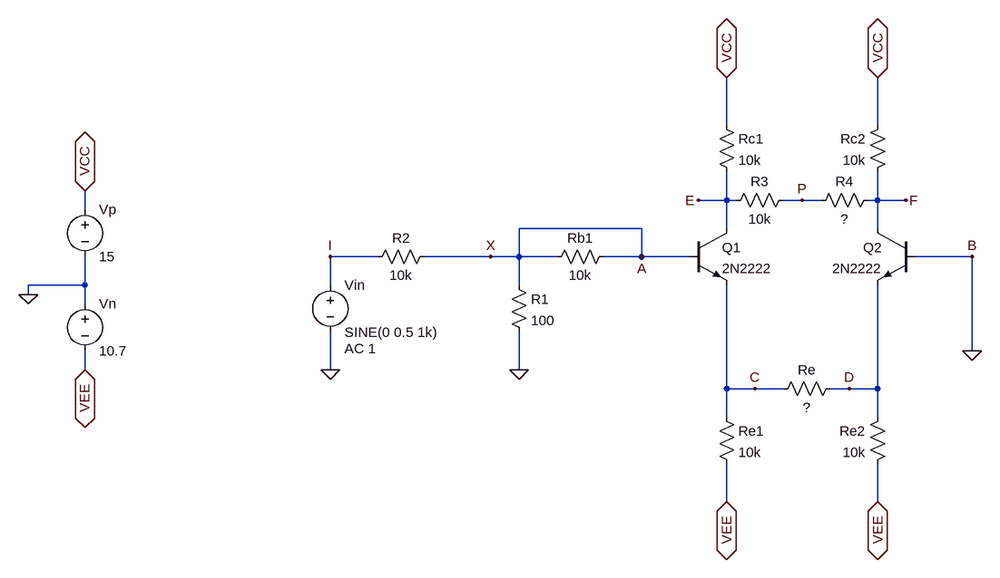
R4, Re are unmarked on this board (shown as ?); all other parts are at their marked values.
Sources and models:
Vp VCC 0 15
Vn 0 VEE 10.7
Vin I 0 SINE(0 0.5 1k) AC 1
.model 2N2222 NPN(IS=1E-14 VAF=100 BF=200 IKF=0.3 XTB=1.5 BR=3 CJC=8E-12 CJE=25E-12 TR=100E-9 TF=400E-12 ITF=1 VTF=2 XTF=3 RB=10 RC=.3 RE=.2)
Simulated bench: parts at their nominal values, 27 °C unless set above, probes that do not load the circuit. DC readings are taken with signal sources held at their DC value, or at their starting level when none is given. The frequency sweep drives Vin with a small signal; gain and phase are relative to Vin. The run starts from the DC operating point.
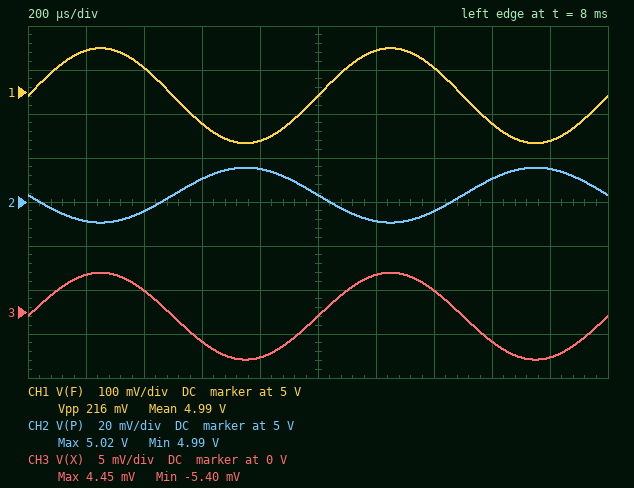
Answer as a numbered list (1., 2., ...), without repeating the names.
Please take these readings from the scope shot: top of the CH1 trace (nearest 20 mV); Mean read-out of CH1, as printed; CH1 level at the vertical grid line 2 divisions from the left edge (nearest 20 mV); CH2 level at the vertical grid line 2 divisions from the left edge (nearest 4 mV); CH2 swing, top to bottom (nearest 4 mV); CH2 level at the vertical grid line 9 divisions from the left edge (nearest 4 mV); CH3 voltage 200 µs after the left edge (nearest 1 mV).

1. 5.10 V
2. 4.99 V
3. 5.06 V
4. 4.996 V
5. 24 mV
6. 5.016 V
7. 4 mV
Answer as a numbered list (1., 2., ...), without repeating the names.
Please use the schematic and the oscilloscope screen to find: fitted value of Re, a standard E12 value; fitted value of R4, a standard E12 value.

1. 180 Ω
2. 12 kΩ
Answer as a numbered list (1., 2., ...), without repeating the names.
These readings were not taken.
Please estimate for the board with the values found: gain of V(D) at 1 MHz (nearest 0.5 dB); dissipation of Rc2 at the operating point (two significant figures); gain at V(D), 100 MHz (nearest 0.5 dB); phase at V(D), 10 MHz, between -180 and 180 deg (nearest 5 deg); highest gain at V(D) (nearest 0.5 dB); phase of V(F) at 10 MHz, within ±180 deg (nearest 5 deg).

1. -59.0 dB
2. 10 mW
3. -62.0 dB
4. -5 deg
5. -59.0 dB
6. -70 deg
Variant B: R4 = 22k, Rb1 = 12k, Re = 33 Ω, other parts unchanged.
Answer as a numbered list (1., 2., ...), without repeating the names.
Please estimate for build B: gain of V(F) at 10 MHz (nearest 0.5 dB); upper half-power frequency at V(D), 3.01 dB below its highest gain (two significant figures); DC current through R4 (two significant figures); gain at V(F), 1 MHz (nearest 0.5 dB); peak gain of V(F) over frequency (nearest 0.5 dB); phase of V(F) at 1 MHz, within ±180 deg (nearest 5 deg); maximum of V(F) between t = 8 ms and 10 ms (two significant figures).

1. -15.0 dB
2. 4.2 MHz
3. 2.0 µA
4. -4.0 dB
5. -3.5 dB
6. -20 deg
7. 5.3 V
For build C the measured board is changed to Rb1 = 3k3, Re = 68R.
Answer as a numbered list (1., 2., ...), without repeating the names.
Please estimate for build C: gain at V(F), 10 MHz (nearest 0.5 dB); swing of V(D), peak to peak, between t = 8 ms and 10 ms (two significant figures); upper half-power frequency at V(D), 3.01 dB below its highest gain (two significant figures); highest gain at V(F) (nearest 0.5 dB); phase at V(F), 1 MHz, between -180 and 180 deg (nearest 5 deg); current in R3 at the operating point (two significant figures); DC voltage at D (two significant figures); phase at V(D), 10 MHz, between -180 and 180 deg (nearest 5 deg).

1. -17.0 dB
2. 2.2 mV
3. 9.7 MHz
4. -7.5 dB
5. -15 deg
6. 1.8 µA
7. -650 mV
8. -10 deg
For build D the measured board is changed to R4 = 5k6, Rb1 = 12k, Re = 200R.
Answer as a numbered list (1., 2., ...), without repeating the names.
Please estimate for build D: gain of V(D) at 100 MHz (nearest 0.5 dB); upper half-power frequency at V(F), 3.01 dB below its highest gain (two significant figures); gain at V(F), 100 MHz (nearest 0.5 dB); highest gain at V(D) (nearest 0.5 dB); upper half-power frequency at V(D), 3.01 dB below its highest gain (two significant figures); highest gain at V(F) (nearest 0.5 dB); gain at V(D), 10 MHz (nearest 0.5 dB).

1. -62.5 dB
2. 6.1 MHz
3. -42.0 dB
4. -59.5 dB
5. 110 MHz
6. -15.5 dB
7. -60.5 dB
